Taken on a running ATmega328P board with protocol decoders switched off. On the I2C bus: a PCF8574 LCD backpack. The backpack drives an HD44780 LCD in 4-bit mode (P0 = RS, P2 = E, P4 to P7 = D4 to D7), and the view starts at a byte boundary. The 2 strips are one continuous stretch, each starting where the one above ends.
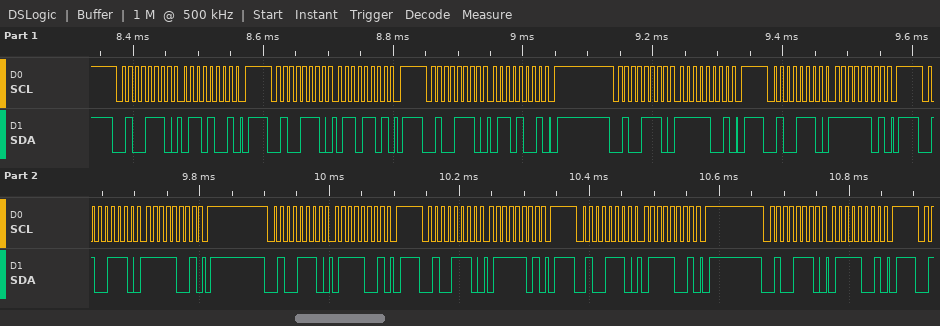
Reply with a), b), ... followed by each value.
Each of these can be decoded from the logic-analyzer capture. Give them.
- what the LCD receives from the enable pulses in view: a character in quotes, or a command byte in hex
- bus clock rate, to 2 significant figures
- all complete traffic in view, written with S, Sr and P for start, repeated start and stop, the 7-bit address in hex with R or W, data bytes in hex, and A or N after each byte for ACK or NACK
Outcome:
a) 'o'
b) 100 kHz
c) S 27W A 69 A P S 27W A 6D A P S 27W A 69 A P S 27W A F9 A P S 27W A FD A P S 27W A F9 A P S 27W A 79 A P S 27W A 7D A P S 27W A 79 A P S 27W A 79 A P
